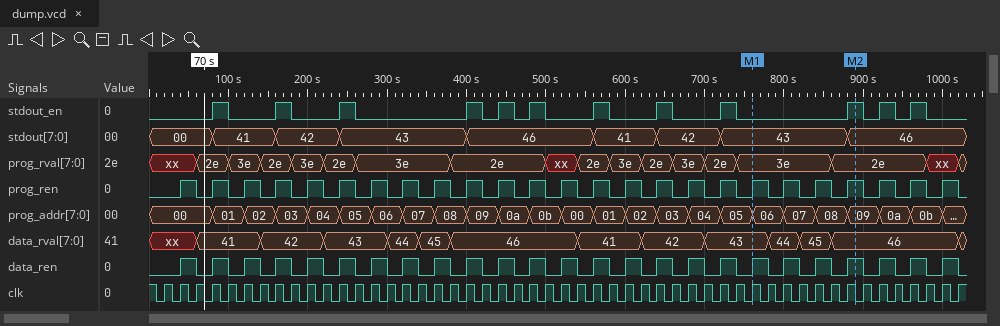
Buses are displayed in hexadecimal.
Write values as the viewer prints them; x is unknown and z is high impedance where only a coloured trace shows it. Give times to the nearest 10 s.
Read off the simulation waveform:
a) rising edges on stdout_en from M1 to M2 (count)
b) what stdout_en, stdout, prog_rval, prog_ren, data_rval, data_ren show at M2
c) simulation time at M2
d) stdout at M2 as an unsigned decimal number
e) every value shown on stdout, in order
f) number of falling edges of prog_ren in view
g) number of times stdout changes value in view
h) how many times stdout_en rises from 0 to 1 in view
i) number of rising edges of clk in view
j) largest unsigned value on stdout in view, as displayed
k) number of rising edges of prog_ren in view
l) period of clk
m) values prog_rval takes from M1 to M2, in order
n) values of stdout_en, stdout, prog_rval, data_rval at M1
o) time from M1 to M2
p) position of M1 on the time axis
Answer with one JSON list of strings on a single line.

["1", "stdout_en=1, stdout=46, prog_rval=2e, prog_ren=1, data_rval=46, data_ren=1", "890 s", "70", "00, 41, 42, 43, 46, 41, 42, 43, 46", "25", "8", "12", "51", "46", "25", "20 s", "3e, 2e", "stdout_en=0, stdout=43, prog_rval=3e, data_rval=43", "130 s", "760 s"]
